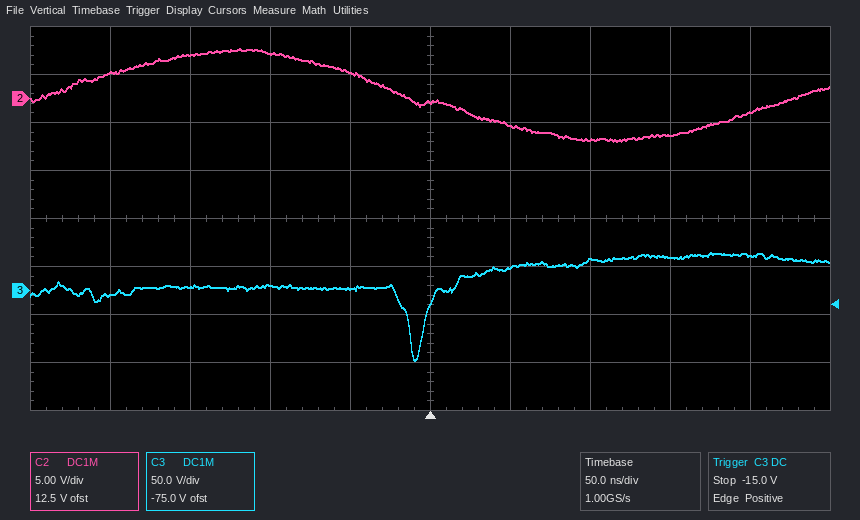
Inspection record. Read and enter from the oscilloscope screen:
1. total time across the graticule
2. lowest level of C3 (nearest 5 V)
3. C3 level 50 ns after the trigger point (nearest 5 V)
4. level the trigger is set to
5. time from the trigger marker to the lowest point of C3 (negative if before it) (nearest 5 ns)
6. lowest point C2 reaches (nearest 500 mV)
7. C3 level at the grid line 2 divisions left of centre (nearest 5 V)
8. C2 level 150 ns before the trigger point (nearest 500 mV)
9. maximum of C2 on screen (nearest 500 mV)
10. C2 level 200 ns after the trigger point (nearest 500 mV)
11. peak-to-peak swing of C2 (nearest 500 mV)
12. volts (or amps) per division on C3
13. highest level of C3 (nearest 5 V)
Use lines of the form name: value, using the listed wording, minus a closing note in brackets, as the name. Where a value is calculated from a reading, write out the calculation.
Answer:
total time across the graticule: 500 ns
lowest level of C3: -75 V
C3 level 50 ns after the trigger point: 25 V
level the trigger is set to: -15.0 V
time from the trigger marker to the lowest point of C3 (negative if before it): -10 ns
lowest point C2 reaches: -4.5 V
C3 level at the grid line 2 divisions left of centre: 5 V
C2 level 150 ns before the trigger point: 4.5 V
maximum of C2 on screen: 5.0 V
C2 level 200 ns after the trigger point: -1.5 V
peak-to-peak swing of C2: 5.0 V − (-4.5 V) = 9.5 V
volts (or amps) per division on C3: 50 V
highest level of C3: 40 V
